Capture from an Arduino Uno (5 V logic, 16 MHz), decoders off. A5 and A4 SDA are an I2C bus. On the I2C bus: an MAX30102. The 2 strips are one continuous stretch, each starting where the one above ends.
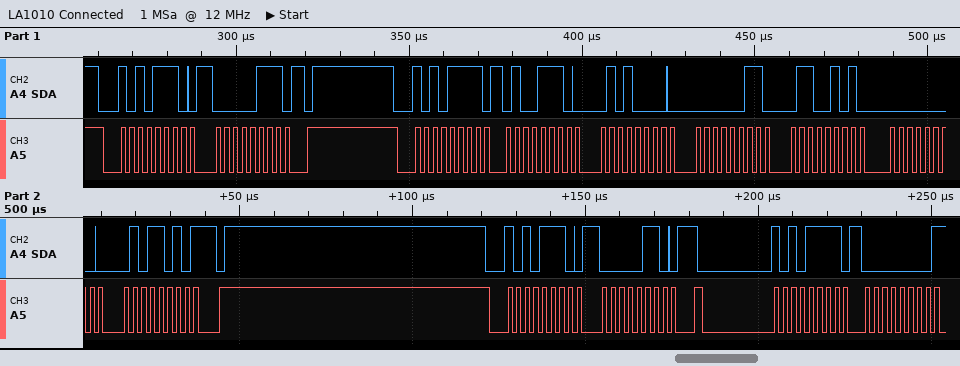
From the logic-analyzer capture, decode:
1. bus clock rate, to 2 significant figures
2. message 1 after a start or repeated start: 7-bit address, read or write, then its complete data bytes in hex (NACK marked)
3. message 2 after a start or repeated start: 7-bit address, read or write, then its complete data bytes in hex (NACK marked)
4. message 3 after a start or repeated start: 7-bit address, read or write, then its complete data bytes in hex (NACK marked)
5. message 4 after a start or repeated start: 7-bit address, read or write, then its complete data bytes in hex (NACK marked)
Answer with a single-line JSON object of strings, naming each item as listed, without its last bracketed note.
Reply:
{"bus clock rate, to 2 significant figures": "400 kHz", "message 1 after a start or repeated start: 7-bit address, read or write, then its complete data bytes in hex": "0x57 write: 07", "message 2 after a start or repeated start: 7-bit address, read or write, then its complete data bytes in hex": "0x57 read: 4E 50 03 65 00 5A NACK", "message 3 after a start or repeated start: 7-bit address, read or write, then its complete data bytes in hex": "0x57 write: 06", "message 4 after a start or repeated start: 7-bit address, read or write, then its complete data bytes in hex": "0x57 read: 00 NACK"}
